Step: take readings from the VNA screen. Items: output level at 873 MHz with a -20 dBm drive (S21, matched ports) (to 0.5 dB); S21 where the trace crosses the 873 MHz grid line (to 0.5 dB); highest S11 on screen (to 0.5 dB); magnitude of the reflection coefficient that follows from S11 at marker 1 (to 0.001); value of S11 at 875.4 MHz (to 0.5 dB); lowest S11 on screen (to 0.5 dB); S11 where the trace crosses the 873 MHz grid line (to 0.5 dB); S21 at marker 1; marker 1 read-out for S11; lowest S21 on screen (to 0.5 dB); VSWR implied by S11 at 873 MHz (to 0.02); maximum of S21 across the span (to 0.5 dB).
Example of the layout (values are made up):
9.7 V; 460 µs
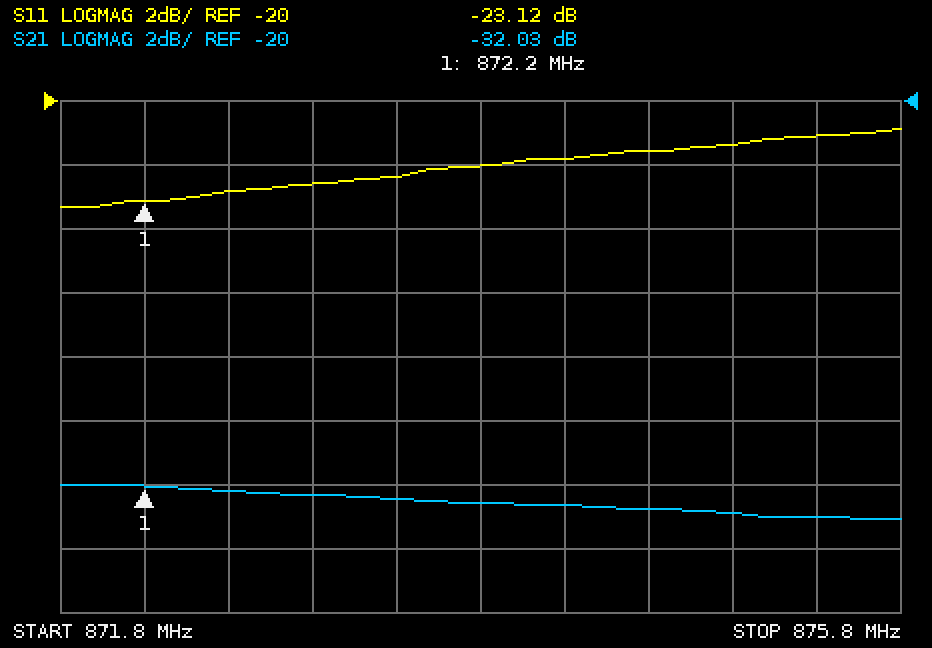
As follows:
-52.5 dBm; -32.5 dB; -21.0 dB; 0.070; -21.0 dB; -23.5 dB; -22.5 dB; -32.03 dB; -23.12 dB; -33.0 dB; 1.16; -32.0 dB
